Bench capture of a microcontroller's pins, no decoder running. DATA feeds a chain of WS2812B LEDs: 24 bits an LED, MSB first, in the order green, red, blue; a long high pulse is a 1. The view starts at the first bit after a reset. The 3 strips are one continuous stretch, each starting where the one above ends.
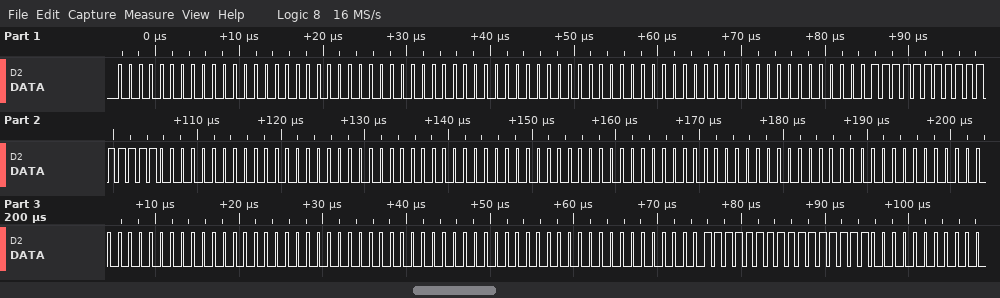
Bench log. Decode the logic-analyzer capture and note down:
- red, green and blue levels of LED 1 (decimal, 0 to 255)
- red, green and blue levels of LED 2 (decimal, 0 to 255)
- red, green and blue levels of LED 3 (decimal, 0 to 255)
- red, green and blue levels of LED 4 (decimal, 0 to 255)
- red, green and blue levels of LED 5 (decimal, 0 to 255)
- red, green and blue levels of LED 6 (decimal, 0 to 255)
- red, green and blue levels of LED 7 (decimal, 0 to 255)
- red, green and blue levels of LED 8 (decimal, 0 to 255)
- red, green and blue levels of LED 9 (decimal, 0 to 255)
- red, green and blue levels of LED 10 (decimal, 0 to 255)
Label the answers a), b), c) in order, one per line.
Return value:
a) 0, 0, 0
b) 0, 0, 0
c) 0, 0, 0
d) 255, 255, 0
e) 0, 0, 0
f) 0, 0, 0
g) 0, 0, 0
h) 0, 0, 0
i) 0, 0, 0
j) 255, 0, 255
